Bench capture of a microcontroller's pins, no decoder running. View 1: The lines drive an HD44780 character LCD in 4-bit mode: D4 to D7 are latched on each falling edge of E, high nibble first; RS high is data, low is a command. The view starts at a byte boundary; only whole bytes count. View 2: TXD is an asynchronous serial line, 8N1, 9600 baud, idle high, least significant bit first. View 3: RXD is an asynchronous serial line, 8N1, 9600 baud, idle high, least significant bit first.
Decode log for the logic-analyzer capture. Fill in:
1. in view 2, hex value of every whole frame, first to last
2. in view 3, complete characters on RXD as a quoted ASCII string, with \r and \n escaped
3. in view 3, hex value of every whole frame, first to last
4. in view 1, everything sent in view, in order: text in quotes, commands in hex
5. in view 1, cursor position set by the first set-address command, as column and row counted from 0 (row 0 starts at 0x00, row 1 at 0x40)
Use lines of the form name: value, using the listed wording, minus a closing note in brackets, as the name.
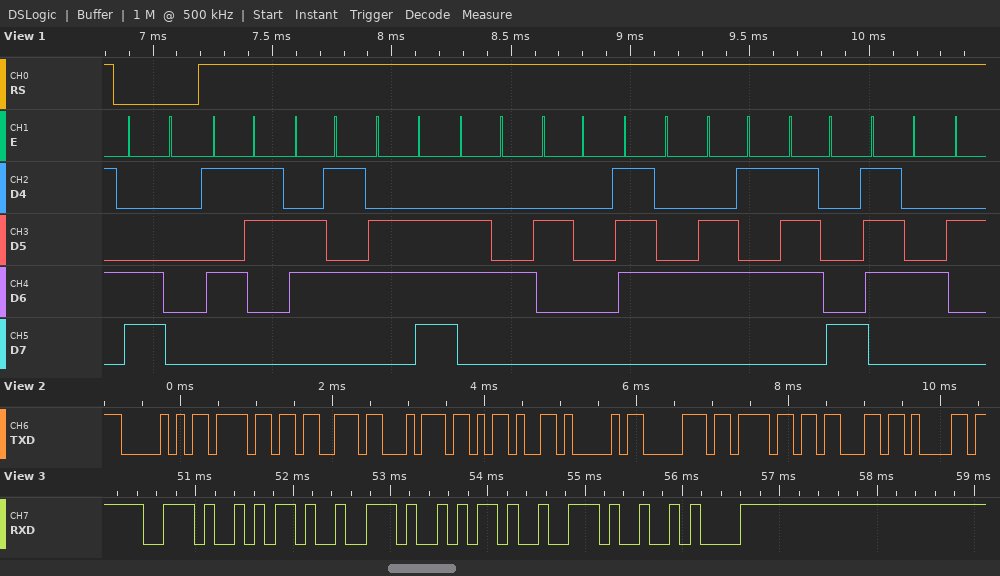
in view 2, hex value of every whole frame, first to last: 50 6F 73 74 2D 41 70 6F 63 61
in view 3, complete characters on RXD as a quoted ASCII string, with \r and \n escaped: ".-.-.\n"
in view 3, hex value of every whole frame, first to last: 2E 2D 2E 2D 2E 0A
in view 1, everything sent in view, in order: text in quotes, commands in hex: 0xC0 "Send text"
in view 1, cursor position set by the first set-address command, as column and row counted from 0: column 0, row 1
